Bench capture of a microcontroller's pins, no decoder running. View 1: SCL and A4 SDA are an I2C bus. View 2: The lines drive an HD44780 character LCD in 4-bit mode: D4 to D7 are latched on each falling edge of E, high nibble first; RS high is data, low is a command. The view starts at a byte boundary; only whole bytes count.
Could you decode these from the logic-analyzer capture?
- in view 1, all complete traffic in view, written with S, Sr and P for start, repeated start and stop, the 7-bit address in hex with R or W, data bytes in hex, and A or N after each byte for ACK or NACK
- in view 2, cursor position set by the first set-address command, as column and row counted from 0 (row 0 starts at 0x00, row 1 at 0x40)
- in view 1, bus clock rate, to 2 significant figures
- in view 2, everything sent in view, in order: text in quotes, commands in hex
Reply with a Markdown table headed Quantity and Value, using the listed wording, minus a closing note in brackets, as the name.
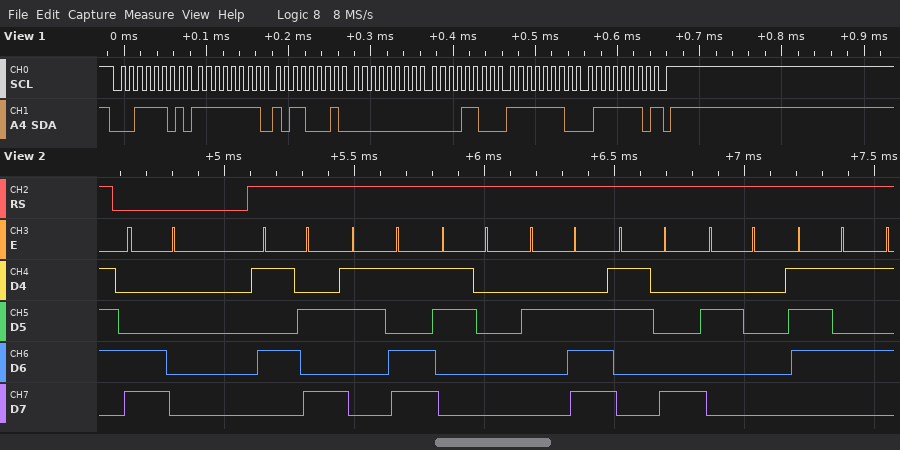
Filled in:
| Quantity | Value |
|---|---|
| in view 1, all complete traffic in view, written with S, Sr and P for start, repeated start and stop, the 7-bit address in hex with R or W, data bytes in hex, and A or N after each byte for ACK or NACK | S 1ER A FF A B1 A 00 A 0C A FE A 7E N P |
| in view 2, cursor position set by the first set-address command, as column and row counted from 0 | column 0, row 1 |
| in view 1, bus clock rate, to 2 significant figures | 100 kHz |
| in view 2, everything sent in view, in order: text in quotes, commands in hex | 0xC0 "Z=0.8 u" |
